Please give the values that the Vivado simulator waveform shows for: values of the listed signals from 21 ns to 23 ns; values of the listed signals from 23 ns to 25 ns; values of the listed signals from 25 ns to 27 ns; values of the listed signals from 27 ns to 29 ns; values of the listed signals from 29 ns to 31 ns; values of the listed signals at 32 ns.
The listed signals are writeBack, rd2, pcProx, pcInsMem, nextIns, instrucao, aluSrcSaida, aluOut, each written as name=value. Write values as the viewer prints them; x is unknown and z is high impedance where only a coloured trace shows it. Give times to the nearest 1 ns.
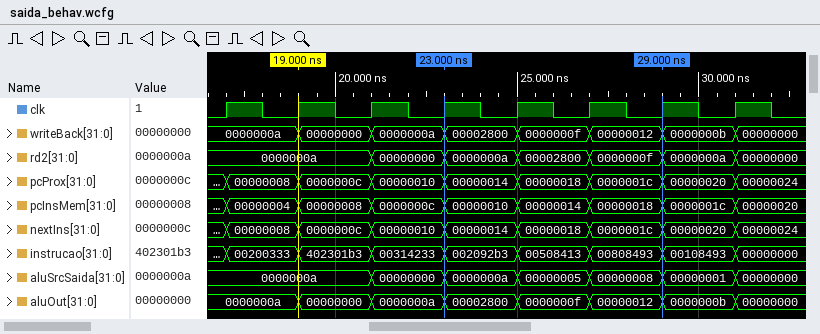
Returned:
writeBack=0000000a, rd2=00000000, pcProx=00000010, pcInsMem=0000000c, nextIns=00000010, instrucao=00314233, aluSrcSaida=00000000, aluOut=0000000a
writeBack=00002800, rd2=0000000a, pcProx=00000014, pcInsMem=00000010, nextIns=00000014, instrucao=002092b3, aluSrcSaida=0000000a, aluOut=00002800
writeBack=0000000f, rd2=00002800, pcProx=00000018, pcInsMem=00000014, nextIns=00000018, instrucao=00508413, aluSrcSaida=00000005, aluOut=0000000f
writeBack=00000012, rd2=0000000f, pcProx=0000001c, pcInsMem=00000018, nextIns=0000001c, instrucao=00808493, aluSrcSaida=00000008, aluOut=00000012
writeBack=0000000b, rd2=0000000a, pcProx=00000020, pcInsMem=0000001c, nextIns=00000020, instrucao=00108493, aluSrcSaida=00000001, aluOut=0000000b
writeBack=00000000, rd2=00000000, pcProx=00000024, pcInsMem=00000020, nextIns=00000024, instrucao=00000000, aluSrcSaida=00000000, aluOut=00000000
